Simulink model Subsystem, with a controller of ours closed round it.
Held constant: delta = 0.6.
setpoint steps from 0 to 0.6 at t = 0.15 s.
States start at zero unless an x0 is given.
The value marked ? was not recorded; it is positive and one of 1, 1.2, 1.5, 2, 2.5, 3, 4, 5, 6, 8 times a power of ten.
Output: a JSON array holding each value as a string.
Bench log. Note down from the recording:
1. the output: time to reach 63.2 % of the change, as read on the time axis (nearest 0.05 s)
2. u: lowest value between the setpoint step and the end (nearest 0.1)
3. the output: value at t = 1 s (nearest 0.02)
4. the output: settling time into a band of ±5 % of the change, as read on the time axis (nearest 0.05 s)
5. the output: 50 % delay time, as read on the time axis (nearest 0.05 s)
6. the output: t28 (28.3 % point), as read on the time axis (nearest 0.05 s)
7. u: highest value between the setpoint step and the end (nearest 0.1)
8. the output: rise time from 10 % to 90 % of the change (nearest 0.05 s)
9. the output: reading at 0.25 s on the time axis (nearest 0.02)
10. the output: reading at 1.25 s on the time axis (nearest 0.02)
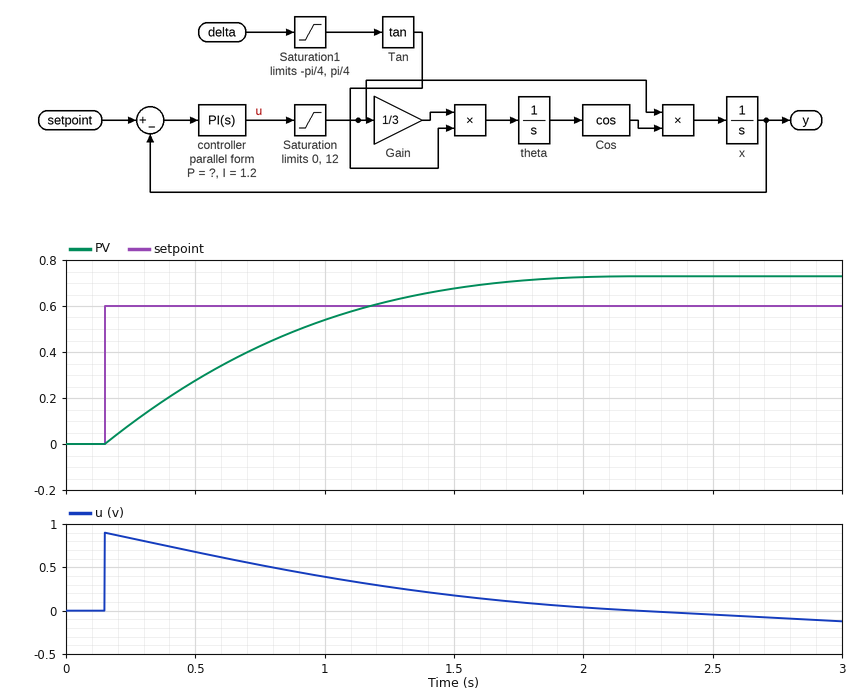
["0.80 s", "-0.1", "0.54", "1.60 s", "0.65 s", "0.40 s", "0.9", "1.15 s", "0.08", "0.62"]
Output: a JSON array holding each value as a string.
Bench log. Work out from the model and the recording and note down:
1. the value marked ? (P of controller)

["1.5"]
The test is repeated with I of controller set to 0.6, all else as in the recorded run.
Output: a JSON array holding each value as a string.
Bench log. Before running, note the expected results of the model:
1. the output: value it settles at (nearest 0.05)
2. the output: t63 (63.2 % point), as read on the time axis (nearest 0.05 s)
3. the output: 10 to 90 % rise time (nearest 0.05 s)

["0.70", "0.85 s", "1.35 s"]
